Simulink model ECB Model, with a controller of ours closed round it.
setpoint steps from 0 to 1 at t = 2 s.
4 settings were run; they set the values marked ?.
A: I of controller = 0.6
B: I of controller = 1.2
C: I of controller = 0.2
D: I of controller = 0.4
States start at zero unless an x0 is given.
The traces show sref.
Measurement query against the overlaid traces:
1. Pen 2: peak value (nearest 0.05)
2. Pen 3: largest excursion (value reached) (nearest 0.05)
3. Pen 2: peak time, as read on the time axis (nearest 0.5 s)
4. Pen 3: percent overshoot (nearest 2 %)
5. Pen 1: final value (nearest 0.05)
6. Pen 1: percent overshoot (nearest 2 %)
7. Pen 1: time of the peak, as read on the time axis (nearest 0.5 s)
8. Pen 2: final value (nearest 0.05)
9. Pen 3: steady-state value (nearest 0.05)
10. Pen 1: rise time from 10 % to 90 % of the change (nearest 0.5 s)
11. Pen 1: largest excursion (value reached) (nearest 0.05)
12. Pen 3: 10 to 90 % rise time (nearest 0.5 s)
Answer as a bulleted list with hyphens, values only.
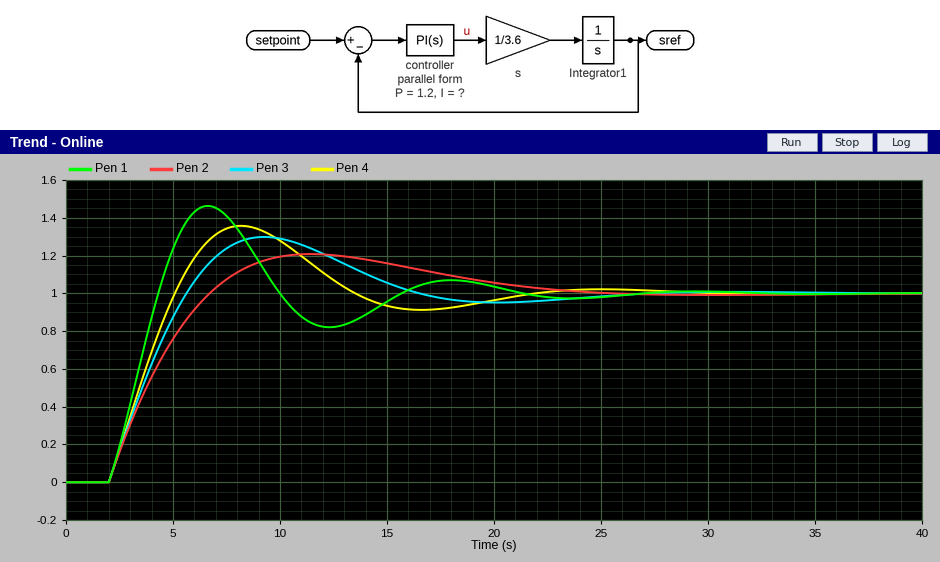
- 1.20
- 1.30
- 11.5 s
- 30 %
- 1.00
- 46 %
- 6.5 s
- 1.00
- 1.00
- 2.0 s
- 1.45
- 3.0 s
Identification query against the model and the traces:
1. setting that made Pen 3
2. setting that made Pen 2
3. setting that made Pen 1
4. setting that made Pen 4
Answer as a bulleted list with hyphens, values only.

- D
- C
- B
- A
